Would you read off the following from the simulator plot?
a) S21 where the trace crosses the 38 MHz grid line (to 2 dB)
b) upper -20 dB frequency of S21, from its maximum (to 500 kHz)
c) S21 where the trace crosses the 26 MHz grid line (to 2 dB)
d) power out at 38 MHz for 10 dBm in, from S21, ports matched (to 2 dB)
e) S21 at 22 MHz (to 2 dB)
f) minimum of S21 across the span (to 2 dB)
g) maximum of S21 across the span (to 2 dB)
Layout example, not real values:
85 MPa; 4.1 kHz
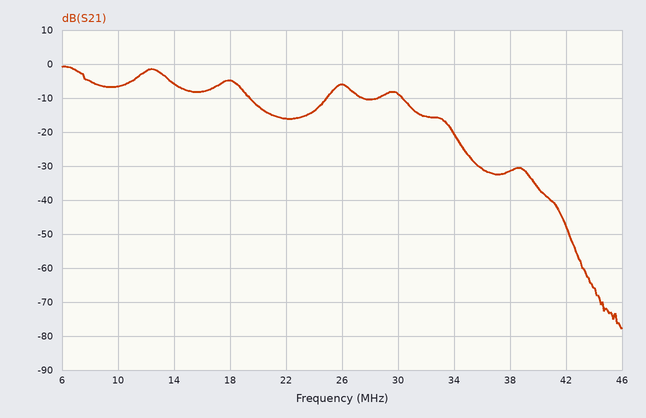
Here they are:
-32 dB; 34.0 MHz; -6 dB; -22 dBm; -16 dB; -78 dB; 0 dB
